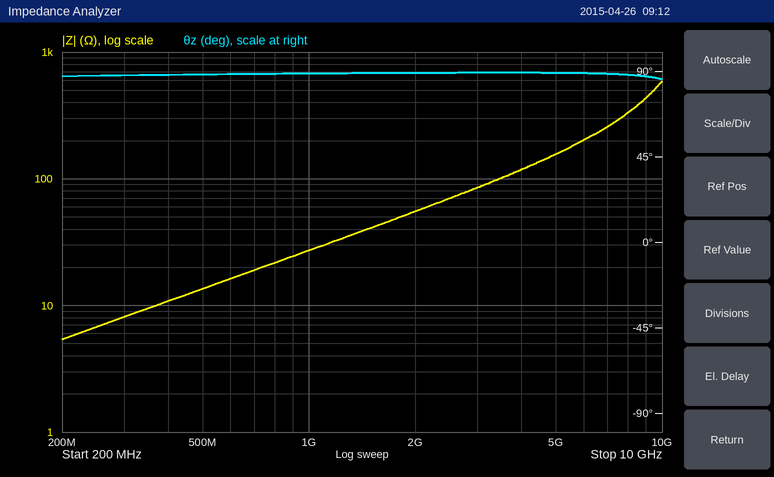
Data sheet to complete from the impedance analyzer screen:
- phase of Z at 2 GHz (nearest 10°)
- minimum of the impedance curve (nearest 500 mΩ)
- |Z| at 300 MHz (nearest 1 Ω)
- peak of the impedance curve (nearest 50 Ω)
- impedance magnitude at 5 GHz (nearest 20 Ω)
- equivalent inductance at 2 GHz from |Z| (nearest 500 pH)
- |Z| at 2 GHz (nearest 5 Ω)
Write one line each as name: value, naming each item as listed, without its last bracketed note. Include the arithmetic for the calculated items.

phase of Z at 2 GHz: 90°
minimum of the impedance curve: 5.5 Ω
|Z| at 300 MHz: 8 Ω
peak of the impedance curve: 600 Ω
impedance magnitude at 5 GHz: 160 Ω
equivalent inductance at 2 GHz from |Z|: L = 55 Ω/(2π × 2 GHz) ≈ 4.38 nH, so 4.5 nH to the nearest 500 pH
|Z| at 2 GHz: 55 Ω
